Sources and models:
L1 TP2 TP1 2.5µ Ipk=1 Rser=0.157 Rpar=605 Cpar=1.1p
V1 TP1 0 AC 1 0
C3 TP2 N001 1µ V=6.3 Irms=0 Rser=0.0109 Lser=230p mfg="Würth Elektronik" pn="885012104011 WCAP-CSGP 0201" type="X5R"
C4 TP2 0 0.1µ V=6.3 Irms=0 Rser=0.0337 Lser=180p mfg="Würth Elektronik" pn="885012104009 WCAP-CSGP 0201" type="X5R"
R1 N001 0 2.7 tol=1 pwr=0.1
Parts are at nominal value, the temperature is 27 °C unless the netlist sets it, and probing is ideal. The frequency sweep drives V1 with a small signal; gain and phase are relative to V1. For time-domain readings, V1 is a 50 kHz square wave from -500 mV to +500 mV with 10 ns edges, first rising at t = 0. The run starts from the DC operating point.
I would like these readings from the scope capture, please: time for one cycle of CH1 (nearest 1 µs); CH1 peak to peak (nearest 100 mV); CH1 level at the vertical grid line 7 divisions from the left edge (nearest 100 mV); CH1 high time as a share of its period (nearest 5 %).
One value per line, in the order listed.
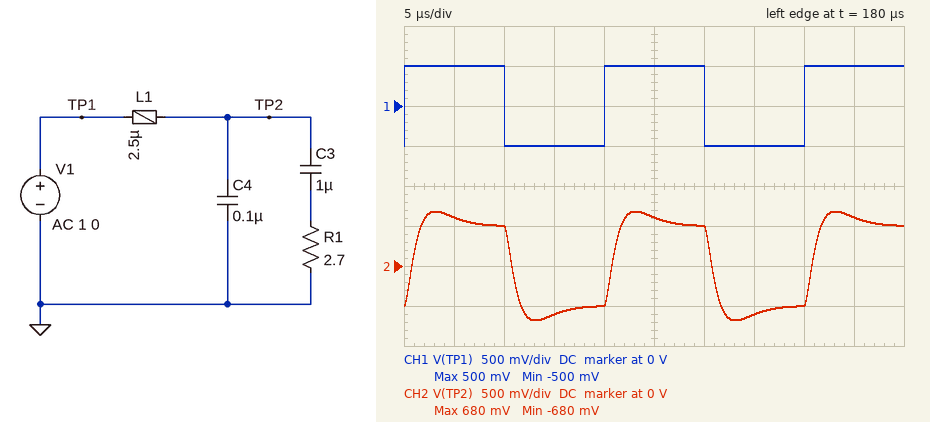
20 µs
1.0 V
-500 mV
50 %
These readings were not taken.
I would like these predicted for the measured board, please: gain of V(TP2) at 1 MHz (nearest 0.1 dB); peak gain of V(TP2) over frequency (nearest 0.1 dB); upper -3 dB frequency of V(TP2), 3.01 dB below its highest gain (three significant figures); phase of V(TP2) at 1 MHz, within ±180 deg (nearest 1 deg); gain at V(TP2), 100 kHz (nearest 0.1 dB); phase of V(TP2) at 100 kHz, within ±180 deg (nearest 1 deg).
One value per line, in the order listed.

-20.8 dB
1.7 dB
201 kHz
-145 deg
1.6 dB
-34 deg
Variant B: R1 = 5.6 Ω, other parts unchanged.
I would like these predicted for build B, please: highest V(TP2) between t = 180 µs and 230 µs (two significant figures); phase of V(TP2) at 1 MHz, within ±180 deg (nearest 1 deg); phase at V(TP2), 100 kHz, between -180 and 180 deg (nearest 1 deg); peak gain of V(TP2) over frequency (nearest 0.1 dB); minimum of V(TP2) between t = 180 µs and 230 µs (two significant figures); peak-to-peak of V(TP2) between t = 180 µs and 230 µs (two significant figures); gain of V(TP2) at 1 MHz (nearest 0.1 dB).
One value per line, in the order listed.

730 mV
-159 deg
-18 deg
2.0 dB
-730 mV
1.5 V
-19.5 dB
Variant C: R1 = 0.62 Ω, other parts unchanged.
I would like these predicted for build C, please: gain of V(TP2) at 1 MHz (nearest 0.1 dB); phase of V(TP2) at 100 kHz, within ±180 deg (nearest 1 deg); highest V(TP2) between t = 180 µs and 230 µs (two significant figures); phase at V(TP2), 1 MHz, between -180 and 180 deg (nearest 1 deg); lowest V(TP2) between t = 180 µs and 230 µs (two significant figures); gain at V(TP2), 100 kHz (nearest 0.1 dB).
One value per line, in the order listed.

-28.9 dB
-79 deg
930 mV
-120 deg
-930 mV
7.1 dB
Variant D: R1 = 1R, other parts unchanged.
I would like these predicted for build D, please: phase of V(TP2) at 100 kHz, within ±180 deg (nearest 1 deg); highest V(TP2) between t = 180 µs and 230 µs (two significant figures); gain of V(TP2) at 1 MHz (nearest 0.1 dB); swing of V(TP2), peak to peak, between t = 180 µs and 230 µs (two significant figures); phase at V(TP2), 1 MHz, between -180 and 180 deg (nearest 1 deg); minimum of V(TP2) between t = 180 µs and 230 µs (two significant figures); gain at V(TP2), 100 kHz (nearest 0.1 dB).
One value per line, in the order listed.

-65 deg
870 mV
-25.6 dB
1.7 V
-124 deg
-870 mV
4.7 dB
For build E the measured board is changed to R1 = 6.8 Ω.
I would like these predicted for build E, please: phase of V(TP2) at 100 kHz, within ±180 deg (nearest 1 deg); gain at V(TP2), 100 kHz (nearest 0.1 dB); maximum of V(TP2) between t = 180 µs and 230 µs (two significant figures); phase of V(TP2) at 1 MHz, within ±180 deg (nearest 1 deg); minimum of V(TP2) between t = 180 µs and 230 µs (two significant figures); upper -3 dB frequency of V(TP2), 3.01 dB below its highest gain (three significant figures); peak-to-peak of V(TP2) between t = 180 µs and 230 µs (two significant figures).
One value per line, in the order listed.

-15 deg
0.9 dB
790 mV
-162 deg
-790 mV
371 kHz
1.6 V
